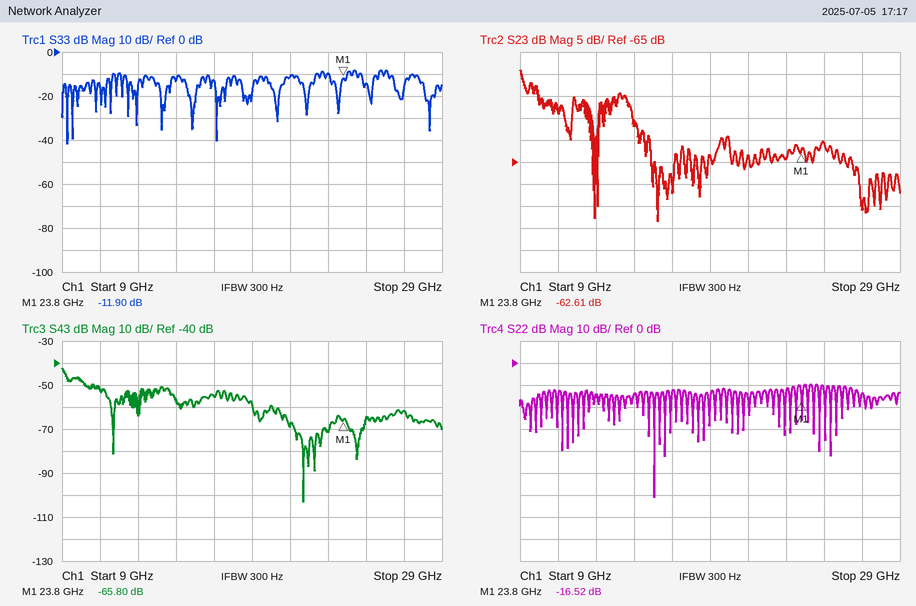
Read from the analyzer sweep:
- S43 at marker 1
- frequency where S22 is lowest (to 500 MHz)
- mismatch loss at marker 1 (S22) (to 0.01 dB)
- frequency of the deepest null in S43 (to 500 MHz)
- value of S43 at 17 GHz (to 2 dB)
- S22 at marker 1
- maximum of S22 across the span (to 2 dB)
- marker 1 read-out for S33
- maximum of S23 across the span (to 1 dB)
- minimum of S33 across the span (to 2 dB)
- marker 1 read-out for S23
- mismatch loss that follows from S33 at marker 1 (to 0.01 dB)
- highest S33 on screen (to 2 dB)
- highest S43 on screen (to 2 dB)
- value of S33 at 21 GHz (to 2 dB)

-65.80 dB
16.0 GHz
0.10 dB
21.5 GHz
-56 dB
-16.52 dB
-10 dB
-11.90 dB
-44 dB
-42 dB
-62.61 dB
0.29 dB
-8 dB
-42 dB
-12 dB
